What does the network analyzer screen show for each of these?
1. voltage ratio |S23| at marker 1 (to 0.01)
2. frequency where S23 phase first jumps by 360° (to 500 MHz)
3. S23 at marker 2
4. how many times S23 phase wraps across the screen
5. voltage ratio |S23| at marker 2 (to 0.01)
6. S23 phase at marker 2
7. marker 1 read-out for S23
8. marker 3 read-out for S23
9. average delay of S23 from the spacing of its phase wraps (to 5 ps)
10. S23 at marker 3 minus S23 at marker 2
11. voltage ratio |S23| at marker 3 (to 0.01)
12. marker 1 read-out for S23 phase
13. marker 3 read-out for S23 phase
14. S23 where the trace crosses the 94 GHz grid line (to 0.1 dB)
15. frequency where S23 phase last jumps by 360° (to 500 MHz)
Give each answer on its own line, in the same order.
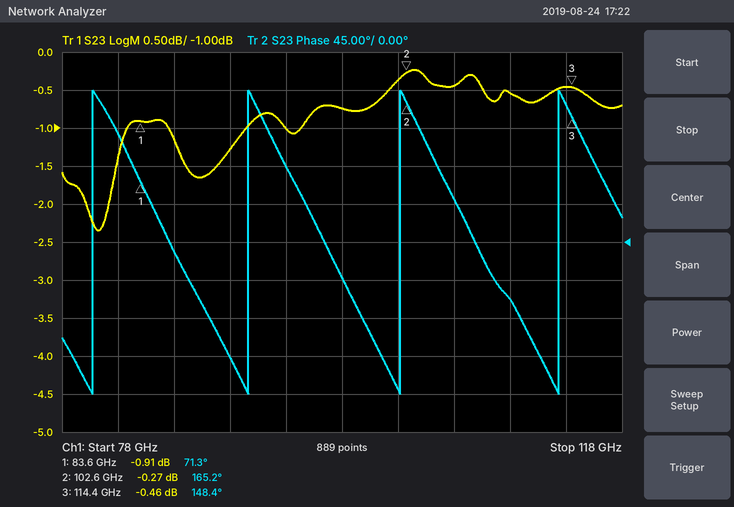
0.90
80.0 GHz
-0.27 dB
4
0.97
165.2°
-0.91 dB
-0.46 dB
90 ps
-0.19 dB
0.95
71.3°
148.4°
-1.0 dB
113.5 GHz
